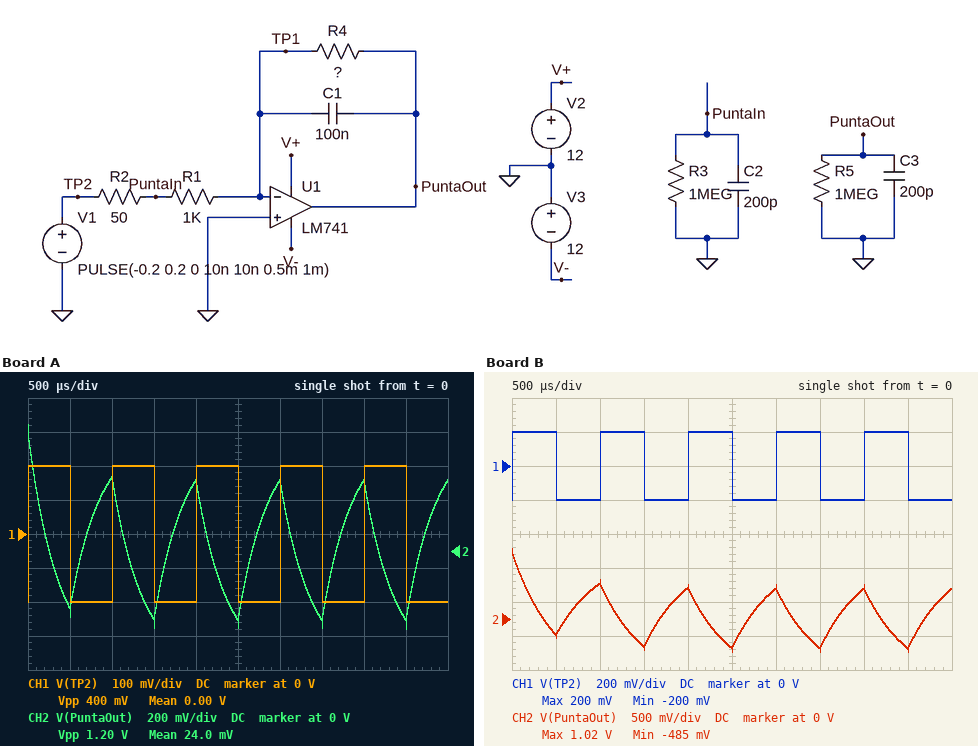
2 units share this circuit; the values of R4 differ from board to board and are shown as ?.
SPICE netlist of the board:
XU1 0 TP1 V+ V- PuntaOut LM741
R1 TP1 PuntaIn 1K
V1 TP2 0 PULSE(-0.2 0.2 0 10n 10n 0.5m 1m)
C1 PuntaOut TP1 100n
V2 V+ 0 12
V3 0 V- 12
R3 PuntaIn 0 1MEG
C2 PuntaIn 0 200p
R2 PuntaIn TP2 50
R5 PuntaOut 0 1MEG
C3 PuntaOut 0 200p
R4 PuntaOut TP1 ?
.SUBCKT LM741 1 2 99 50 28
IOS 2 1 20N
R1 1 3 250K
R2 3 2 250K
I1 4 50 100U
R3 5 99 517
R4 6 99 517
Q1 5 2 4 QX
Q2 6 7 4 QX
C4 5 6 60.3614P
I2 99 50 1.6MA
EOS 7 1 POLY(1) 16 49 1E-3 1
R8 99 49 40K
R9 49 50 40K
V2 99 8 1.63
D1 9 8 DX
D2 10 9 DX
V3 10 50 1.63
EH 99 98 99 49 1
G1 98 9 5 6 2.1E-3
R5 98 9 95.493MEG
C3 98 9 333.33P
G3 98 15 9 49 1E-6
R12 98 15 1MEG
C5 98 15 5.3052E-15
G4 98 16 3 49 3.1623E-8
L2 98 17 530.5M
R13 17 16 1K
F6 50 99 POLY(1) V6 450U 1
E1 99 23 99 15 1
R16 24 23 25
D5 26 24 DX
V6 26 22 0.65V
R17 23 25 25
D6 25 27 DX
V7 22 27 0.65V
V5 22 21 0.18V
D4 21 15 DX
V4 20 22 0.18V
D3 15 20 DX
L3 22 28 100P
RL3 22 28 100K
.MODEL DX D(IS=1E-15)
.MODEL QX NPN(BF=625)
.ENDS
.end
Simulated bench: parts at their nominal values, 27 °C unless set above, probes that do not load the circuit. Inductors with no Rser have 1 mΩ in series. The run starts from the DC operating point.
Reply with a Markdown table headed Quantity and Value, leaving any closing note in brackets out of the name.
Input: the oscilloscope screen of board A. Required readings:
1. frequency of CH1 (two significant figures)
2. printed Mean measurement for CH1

| Quantity | Value |
|---|---|
| frequency of CH1 | 1.0 kHz |
| printed Mean measurement for CH1 | 0.00 V |
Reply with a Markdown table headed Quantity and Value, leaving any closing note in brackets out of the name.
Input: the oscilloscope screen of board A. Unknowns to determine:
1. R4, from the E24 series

| Quantity | Value |
|---|---|
| R4, from the E24 series | 3.6 kΩ |
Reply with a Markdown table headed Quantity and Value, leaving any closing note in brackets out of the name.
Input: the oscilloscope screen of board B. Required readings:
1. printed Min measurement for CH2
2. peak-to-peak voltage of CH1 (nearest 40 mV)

| Quantity | Value |
|---|---|
| printed Min measurement for CH2 | -485 mV |
| peak-to-peak voltage of CH1 | 400 mV |
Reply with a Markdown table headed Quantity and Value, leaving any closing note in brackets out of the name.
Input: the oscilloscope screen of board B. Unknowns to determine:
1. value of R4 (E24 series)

| Quantity | Value |
|---|---|
| value of R4 | 5.1 kΩ |
